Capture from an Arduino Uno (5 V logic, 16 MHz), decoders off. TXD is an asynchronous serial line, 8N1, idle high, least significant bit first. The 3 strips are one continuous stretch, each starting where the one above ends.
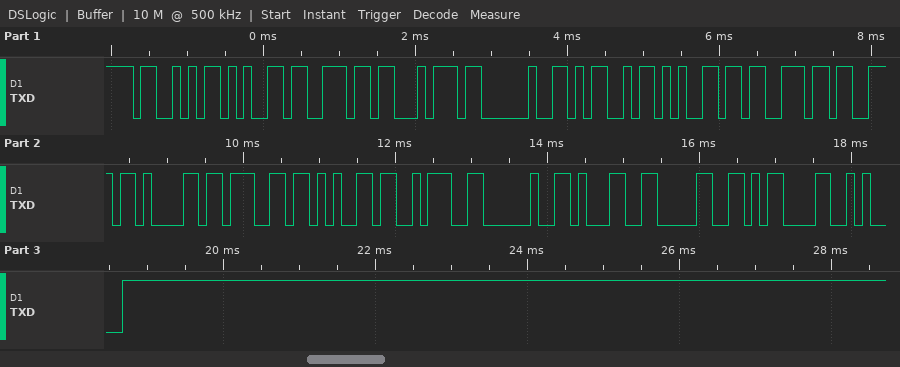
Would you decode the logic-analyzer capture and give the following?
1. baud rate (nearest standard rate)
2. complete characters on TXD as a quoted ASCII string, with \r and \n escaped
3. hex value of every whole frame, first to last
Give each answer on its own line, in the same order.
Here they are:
9600 baud
"Sent Message: 10\r\n"
53 65 6E 74 20 4D 65 73 73 61 67 65 3A 20 31 30 0D 0A
